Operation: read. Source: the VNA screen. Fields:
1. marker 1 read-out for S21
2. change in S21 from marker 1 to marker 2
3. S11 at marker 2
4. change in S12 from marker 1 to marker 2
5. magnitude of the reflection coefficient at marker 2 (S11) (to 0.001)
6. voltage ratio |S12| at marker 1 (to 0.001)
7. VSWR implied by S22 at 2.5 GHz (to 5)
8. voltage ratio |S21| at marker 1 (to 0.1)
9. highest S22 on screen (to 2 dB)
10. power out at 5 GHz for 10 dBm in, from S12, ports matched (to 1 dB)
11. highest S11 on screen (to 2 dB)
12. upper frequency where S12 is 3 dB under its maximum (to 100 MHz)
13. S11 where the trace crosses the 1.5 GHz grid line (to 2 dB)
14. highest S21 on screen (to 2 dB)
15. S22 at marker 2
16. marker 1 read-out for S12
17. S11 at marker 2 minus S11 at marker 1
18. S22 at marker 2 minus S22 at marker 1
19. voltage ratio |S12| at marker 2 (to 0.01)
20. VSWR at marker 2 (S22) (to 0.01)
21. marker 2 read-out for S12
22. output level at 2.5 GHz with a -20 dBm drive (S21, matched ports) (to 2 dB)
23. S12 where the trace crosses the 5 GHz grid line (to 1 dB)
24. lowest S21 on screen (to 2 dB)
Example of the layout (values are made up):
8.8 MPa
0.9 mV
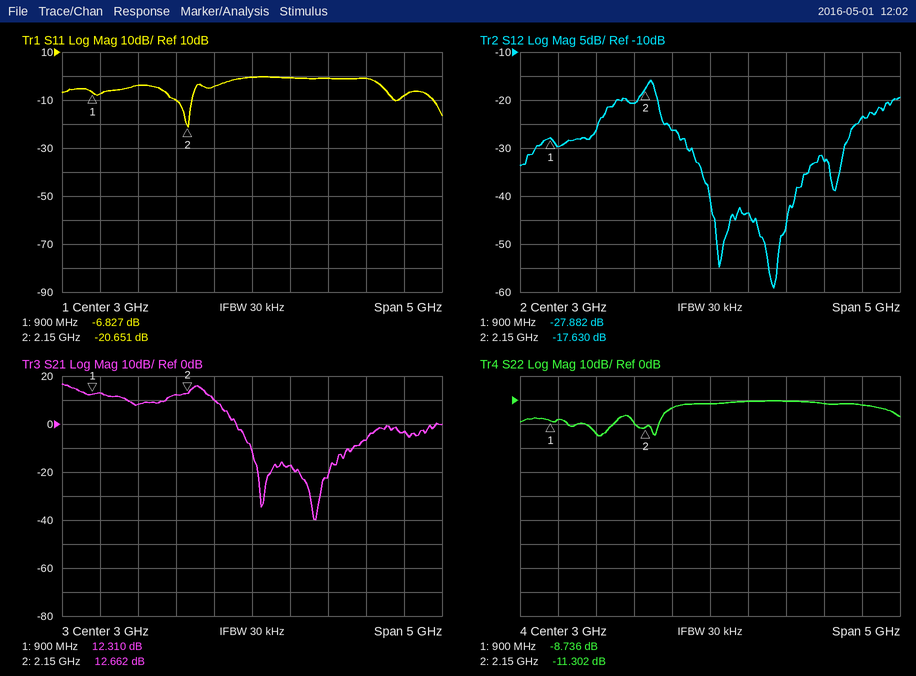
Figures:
12.310 dB
0.352 dB
-20.651 dB
10.252 dB
0.093
0.040
5
4.1
0 dB
-14 dBm
0 dB
2.3 GHz
-4 dB
16 dB
-11.302 dB
-27.882 dB
-13.824 dB
-2.566 dB
0.13
1.75
-17.630 dB
-10 dBm
-24 dB
-40 dB
